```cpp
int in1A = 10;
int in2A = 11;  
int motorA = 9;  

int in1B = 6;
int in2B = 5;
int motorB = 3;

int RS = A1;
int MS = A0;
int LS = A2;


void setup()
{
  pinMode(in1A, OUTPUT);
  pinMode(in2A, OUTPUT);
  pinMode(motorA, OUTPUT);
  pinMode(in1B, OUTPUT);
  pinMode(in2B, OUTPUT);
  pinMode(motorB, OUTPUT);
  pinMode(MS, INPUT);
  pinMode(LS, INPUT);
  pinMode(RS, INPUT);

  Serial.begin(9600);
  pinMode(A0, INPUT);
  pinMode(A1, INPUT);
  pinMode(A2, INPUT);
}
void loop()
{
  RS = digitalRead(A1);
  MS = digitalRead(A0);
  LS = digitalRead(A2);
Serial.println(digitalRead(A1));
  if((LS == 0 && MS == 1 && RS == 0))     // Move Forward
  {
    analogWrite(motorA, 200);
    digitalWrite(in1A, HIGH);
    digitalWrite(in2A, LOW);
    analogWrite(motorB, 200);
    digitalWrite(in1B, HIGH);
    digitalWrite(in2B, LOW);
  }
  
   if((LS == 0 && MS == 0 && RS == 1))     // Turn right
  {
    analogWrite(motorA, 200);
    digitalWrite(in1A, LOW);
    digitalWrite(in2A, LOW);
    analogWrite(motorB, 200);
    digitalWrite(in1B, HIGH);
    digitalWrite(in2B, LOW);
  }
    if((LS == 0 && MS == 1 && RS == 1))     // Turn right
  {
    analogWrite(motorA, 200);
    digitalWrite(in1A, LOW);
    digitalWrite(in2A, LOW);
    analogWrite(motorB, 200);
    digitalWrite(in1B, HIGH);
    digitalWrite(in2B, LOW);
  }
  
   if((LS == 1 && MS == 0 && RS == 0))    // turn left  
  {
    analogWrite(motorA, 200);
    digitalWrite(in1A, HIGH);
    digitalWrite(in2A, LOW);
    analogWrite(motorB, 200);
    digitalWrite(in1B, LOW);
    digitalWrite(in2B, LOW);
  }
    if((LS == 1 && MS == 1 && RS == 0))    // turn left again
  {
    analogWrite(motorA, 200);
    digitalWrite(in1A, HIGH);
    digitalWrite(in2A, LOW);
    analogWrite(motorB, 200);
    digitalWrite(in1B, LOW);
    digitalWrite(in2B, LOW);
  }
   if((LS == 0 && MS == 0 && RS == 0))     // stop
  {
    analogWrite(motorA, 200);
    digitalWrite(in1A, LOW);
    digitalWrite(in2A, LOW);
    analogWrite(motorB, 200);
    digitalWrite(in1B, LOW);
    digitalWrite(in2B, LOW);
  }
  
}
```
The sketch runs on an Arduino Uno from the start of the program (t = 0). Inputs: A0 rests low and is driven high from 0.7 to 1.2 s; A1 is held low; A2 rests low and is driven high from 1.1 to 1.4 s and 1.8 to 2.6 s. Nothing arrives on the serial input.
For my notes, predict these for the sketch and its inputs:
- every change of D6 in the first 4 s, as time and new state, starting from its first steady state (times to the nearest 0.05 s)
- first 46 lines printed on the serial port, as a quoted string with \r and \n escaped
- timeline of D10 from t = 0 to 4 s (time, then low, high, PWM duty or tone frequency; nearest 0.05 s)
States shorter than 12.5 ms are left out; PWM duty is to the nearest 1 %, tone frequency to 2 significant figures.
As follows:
0 s low; 0.7 s high; 1.1 s low
"0\r\n0\r\n0\r\n0\r\n0\r\n0\r\n0\r\n0\r\n0\r\n0\r\n0\r\n0\r\n0\r\n0\r\n0\r\n0\r\n0\r\n0\r\n0\r\n0\r\n0\r\n0\r\n0\r\n0\r\n0\r\n0\r\n0\r\n0\r\n0\r\n0\r\n0\r\n0\r\n0\r\n0\r\n0\r\n0\r\n0\r\n0\r\n0\r\n0\r\n0\r\n0\r\n0\r\n0\r\n0\r\n0\r\n"
0 s low; 0.7 s high; 1.4 s low; 1.8 s high; 2.6 s low
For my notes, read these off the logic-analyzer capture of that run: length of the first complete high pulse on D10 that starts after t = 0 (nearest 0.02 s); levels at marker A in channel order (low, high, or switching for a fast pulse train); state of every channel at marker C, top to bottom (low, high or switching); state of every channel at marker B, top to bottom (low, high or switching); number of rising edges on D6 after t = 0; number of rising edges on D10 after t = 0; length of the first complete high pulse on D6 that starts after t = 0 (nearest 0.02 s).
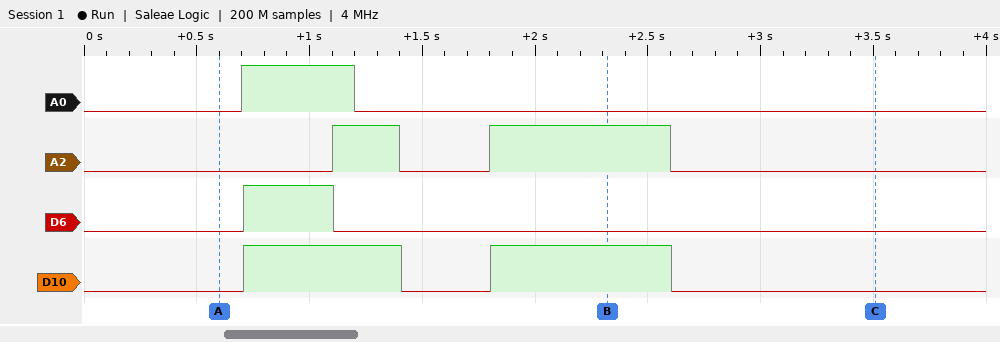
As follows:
0.70 s
A0 low, A2 low, D6 low, D10 low
A0 low, A2 low, D6 low, D10 low
A0 low, A2 high, D6 low, D10 high
1
2
0.40 s
